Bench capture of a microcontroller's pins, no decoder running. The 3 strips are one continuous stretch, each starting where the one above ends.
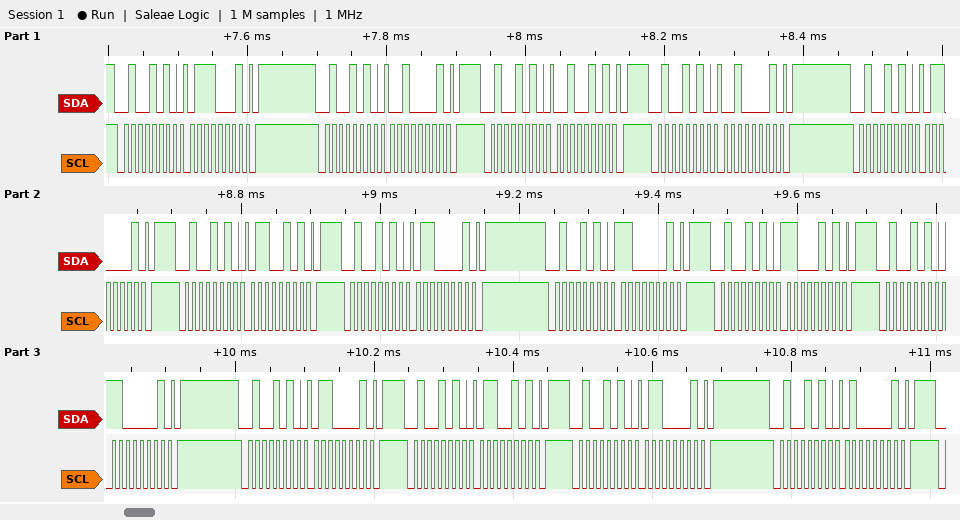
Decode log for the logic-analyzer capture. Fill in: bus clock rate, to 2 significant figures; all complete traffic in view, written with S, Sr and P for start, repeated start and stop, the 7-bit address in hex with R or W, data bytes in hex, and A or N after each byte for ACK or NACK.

100 kHz
S 25W A 71 A P S 25W A 21 A P S 25W A 25 A P S 25W A 21 A P S 25W A 61 A P S 25W A 65 A P S 25W A 61 A P S 25W A C1 A P S 25W A C5 A P S 25W A C1 A P S 25W A 61 A P S 25W A 65 A P S 25W A 61 A P S 25W A 41 A P
